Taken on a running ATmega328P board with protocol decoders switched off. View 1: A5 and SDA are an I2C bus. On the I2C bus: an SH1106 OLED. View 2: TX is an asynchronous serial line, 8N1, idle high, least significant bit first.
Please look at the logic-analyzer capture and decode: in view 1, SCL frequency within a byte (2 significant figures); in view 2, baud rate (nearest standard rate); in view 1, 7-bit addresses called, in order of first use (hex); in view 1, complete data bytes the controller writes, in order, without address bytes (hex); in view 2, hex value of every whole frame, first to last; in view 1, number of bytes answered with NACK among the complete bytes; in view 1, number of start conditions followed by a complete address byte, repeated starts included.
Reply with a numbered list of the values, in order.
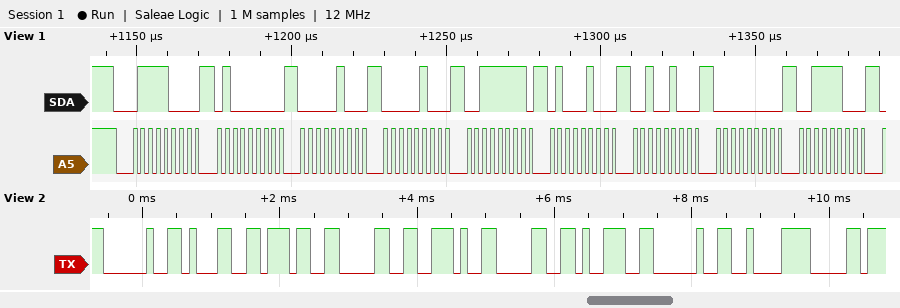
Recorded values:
1. 400 kHz
2. 9600 baud
3. 0x3C
4. 40 04 04 3F 44 24 00 3C
5. 0x20 0x31 0x37 0x30 0x2E 0x30 0x39 0x20 0xC2 0xB0
6. 0
7. 1
